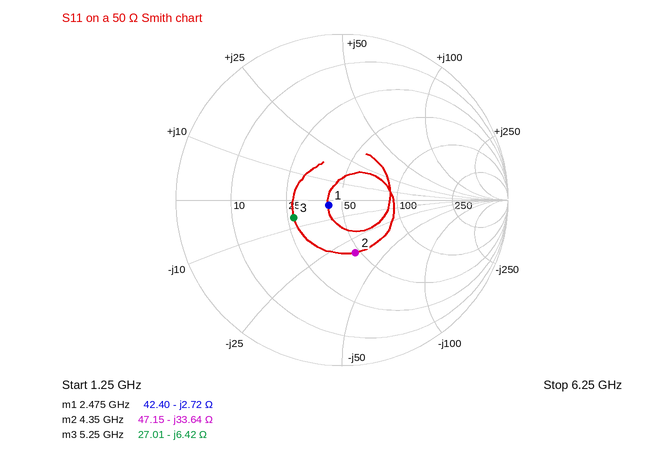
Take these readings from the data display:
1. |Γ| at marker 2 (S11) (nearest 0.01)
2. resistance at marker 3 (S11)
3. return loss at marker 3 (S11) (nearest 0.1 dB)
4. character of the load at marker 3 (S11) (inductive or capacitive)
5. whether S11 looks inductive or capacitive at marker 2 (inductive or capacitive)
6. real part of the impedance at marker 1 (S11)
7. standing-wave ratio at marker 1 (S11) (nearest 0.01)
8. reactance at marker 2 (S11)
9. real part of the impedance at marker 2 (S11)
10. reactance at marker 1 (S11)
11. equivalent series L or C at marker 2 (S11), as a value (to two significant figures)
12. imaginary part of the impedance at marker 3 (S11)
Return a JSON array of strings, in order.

["0.33", "27.01 Ω", "10.2 dB", "capacitive", "capacitive", "42.40 Ω", "1.19", "-33.64 Ω", "47.15 Ω", "-2.72 Ω", "1.1 pF", "-6.42 Ω"]
